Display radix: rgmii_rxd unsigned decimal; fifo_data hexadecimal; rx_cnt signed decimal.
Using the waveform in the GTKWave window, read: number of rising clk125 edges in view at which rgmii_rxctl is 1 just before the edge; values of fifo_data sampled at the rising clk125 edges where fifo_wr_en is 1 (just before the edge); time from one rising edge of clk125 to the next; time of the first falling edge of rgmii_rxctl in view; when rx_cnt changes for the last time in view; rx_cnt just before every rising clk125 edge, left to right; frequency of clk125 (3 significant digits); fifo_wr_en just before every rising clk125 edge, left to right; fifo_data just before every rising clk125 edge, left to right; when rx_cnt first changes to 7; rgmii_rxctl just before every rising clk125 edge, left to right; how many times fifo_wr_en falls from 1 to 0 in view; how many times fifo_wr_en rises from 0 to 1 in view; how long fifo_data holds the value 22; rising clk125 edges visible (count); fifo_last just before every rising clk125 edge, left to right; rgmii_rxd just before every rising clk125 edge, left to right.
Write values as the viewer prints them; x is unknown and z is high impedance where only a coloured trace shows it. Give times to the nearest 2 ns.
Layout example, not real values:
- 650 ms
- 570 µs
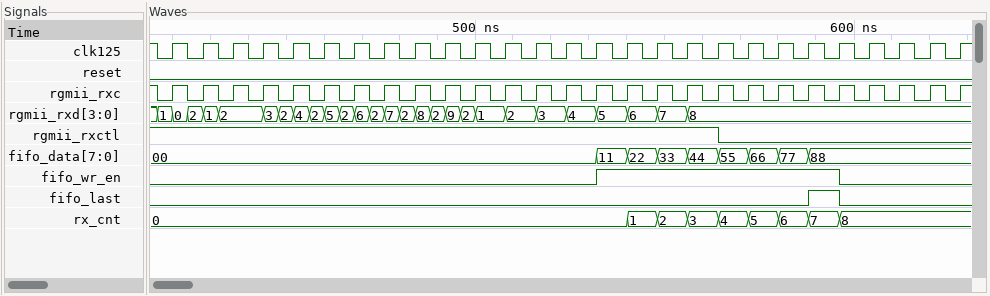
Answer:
- 19
- 11, 22, 33, 44, 55, 66, 77, 88
- 8 ns
- 564 ns
- 596 ns
- 0, 0, 0, 0, 0, 0, 0, 0, 0, 0, 0, 0, 0, 0, 0, 0, 1, 2, 3, 4, 5, 6, 7, 8, 8, 8, 8
- 125 MHz
- 0 0 0 0 0 0 0 0 0 0 0 0 0 0 0 1 1 1 1 1 1 1 1 0 0 0 0
- 00, 00, 00, 00, 00, 00, 00, 00, 00, 00, 00, 00, 00, 00, 00, 11, 22, 33, 44, 55, 66, 77, 88, 88, 88, 88, 88
- 588 ns
- 1 1 1 1 1 1 1 1 1 1 1 1 1 1 1 1 1 1 1 0 0 0 0 0 0 0 0
- 1
- 1
- 8 ns
- 27
- 0 0 0 0 0 0 0 0 0 0 0 0 0 0 0 0 0 0 0 0 0 0 1 0 0 0 0
- 1, 2, 2, 2, 2, 2, 2, 2, 2, 2, 2, 1, 2, 3, 4, 5, 6, 7, 8, 8, 8, 8, 8, 8, 8, 8, 8
